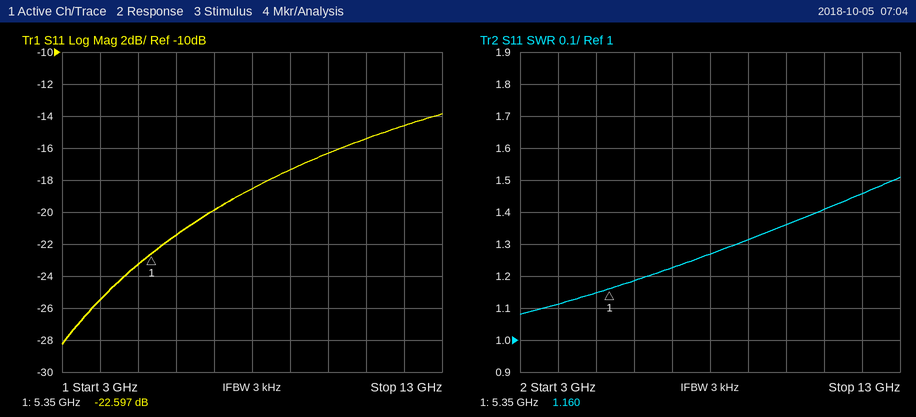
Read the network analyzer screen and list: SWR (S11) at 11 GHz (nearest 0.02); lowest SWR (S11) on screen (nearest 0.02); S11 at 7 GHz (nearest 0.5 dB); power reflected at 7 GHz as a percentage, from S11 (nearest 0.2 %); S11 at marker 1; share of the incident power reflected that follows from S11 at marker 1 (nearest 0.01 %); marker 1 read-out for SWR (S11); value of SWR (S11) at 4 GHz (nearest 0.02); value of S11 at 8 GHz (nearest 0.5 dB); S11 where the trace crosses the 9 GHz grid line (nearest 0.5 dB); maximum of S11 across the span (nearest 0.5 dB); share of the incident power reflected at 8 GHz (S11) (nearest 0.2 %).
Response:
1.40
1.08
-20.0 dB
1.0 %
-22.597 dB
0.55 %
1.160
1.12
-18.5 dB
-17.5 dB
-14.0 dB
1.4 %
